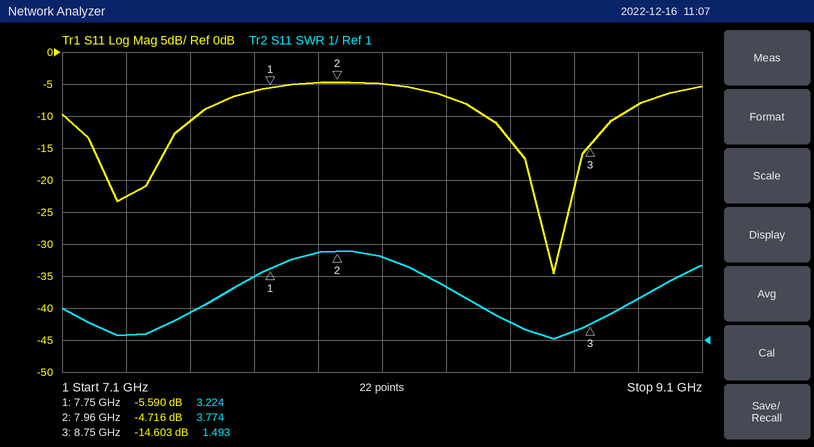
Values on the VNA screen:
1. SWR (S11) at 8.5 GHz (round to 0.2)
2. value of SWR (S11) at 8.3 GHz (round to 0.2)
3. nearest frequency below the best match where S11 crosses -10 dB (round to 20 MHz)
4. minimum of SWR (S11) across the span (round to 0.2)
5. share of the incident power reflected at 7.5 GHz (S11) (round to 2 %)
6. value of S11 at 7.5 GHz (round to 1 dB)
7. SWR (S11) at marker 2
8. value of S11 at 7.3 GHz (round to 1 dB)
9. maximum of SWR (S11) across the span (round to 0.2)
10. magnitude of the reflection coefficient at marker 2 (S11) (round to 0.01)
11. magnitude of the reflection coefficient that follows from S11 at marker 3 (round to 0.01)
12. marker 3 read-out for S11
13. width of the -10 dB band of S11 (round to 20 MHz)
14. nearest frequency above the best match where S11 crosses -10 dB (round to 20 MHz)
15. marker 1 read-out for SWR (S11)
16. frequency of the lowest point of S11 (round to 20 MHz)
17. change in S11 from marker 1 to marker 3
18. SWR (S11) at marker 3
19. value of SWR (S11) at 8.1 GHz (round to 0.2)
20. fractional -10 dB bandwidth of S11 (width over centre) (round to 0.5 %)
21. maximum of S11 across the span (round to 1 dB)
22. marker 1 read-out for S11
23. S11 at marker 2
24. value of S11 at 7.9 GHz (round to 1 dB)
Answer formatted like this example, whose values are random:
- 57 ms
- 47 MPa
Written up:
- 1.6
- 2.6
- 8.42 GHz
- 1.0
- 8 %
- -11 dB
- 3.774
- -23 dB
- 3.8
- 0.58
- 0.19
- -14.603 dB
- 420 MHz
- 8.84 GHz
- 3.224
- 8.64 GHz
- -9.013 dB
- 1.493
- 3.6
- 5.0 %
- -5 dB
- -5.590 dB
- -4.716 dB
- -5 dB
